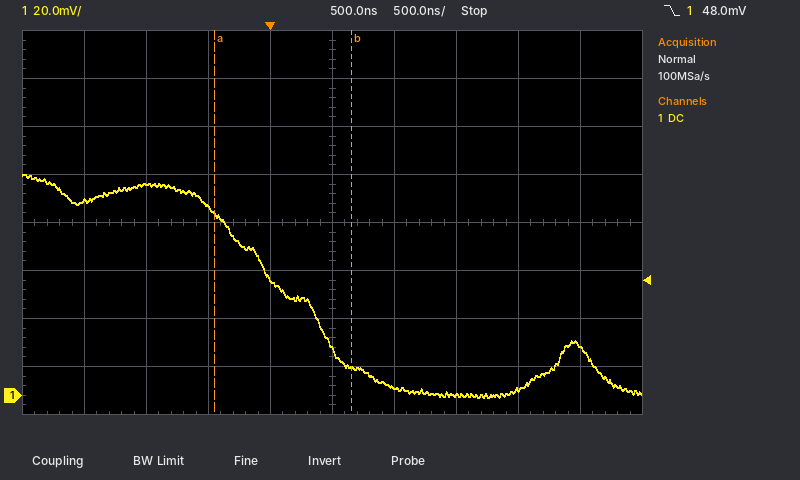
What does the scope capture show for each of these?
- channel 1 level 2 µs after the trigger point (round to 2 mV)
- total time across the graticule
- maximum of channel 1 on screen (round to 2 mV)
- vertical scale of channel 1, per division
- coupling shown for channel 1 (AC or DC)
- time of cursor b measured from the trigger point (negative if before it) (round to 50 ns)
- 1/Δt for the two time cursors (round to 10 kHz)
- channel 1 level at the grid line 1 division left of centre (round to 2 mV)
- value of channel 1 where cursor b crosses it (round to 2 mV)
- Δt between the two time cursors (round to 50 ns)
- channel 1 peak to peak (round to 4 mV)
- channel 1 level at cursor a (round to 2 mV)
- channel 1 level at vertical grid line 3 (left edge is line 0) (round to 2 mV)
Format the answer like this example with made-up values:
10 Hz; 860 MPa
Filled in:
2 mV; 5 µs; 92 mV; 20 mV; DC; +650 ns; 910 kHz; 48 mV; 12 mV; 1.10 µs; 92 mV; 76 mV; 78 mV
